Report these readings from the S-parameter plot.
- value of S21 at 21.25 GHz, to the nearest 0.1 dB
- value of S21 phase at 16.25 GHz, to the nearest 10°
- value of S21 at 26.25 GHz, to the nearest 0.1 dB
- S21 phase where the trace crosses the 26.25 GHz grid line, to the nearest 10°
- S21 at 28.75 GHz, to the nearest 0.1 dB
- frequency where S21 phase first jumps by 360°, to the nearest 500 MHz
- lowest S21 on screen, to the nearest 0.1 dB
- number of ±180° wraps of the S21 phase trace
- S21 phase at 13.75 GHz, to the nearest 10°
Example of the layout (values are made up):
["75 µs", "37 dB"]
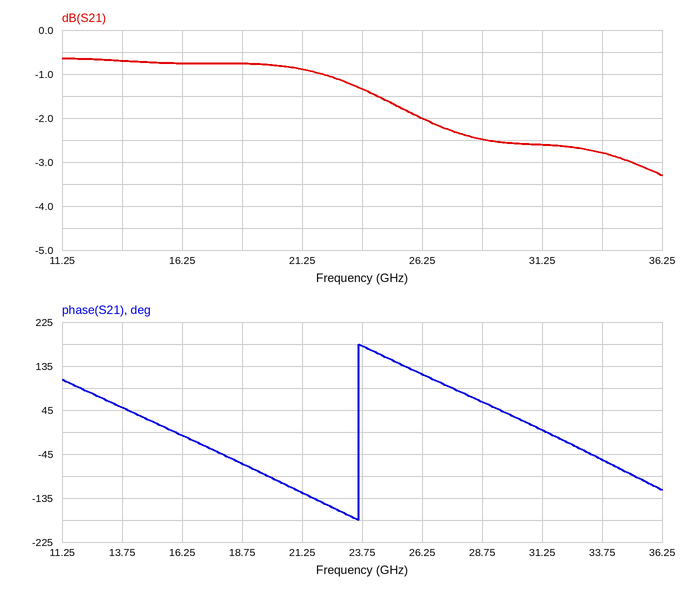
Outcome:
["-0.9 dB", "-10°", "-2.0 dB", "120°", "-2.5 dB", "23.5 GHz", "-3.3 dB", "1", "50°"]
